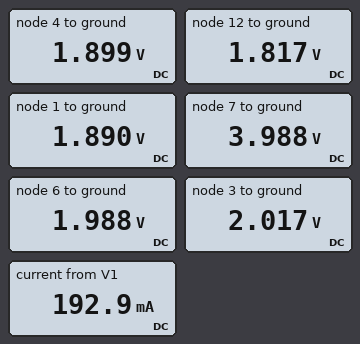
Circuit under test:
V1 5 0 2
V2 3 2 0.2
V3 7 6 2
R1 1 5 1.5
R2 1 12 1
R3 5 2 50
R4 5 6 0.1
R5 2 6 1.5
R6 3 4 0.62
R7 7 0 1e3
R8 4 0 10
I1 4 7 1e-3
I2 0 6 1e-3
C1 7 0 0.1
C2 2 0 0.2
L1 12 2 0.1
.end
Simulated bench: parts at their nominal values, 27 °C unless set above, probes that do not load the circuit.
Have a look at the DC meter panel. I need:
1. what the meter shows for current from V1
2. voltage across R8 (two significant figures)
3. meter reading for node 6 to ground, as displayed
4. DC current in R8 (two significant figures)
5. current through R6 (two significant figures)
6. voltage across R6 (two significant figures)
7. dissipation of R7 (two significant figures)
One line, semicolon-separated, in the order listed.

192.9 mA; 1.9 V; 1.988 V; 190 mA; 190 mA; 120 mV; 16 mW
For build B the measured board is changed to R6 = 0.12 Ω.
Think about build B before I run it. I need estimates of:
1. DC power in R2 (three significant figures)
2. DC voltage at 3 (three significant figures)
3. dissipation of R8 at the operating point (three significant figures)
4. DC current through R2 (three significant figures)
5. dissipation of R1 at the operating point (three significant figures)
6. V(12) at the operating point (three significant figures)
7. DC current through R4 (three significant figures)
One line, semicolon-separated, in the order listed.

5.84 mW; 2.01 V; 394 mW; 76.4 mA; 8.76 mW; 1.81 V; 121 mA
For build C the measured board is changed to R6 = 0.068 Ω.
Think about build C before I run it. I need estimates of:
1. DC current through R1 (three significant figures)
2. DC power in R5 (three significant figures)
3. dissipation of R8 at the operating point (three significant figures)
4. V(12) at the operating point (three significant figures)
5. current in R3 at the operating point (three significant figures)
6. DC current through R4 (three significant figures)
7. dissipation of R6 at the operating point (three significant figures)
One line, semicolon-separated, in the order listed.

76.8 mA; 21.5 mW; 398 mW; 1.81 V; 3.84 mA; 122 mA; 2.73 mW
